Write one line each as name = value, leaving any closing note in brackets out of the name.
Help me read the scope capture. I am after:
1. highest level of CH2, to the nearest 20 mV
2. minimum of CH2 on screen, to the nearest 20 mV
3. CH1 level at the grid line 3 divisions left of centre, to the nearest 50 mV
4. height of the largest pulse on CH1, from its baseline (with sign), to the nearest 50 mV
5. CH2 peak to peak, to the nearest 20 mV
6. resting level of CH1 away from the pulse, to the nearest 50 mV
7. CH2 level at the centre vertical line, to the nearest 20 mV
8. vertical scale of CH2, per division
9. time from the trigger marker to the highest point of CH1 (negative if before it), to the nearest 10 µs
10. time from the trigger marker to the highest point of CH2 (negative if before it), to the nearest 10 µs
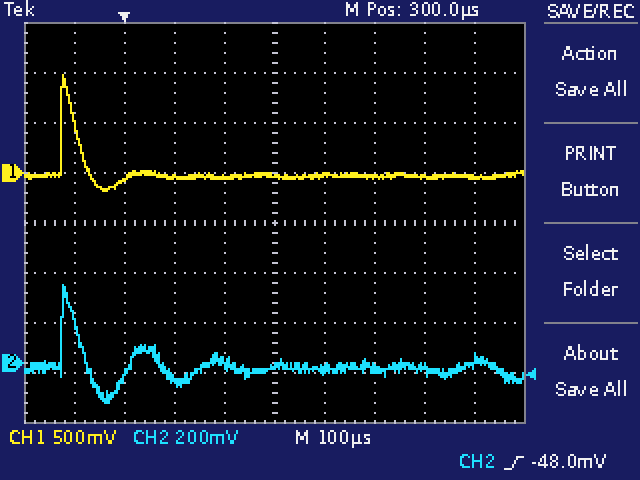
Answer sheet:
highest level of CH2, to the nearest 20 mV = 320 mV
minimum of CH2 on screen, to the nearest 20 mV = -160 mV
CH1 level at the grid line 3 divisions left of centre, to the nearest 50 mV = -50 mV
height of the largest pulse on CH1, from its baseline (with sign), to the nearest 50 mV = +1.00 V
CH2 peak to peak, to the nearest 20 mV = 480 mV
resting level of CH1 away from the pulse, to the nearest 50 mV = -50 mV
CH2 level at the centre vertical line, to the nearest 20 mV = -20 mV
vertical scale of CH2, per division = 200 mV
time from the trigger marker to the highest point of CH1 (negative if before it), to the nearest 10 µs = -120 µs
time from the trigger marker to the highest point of CH2 (negative if before it), to the nearest 10 µs = -120 µs
